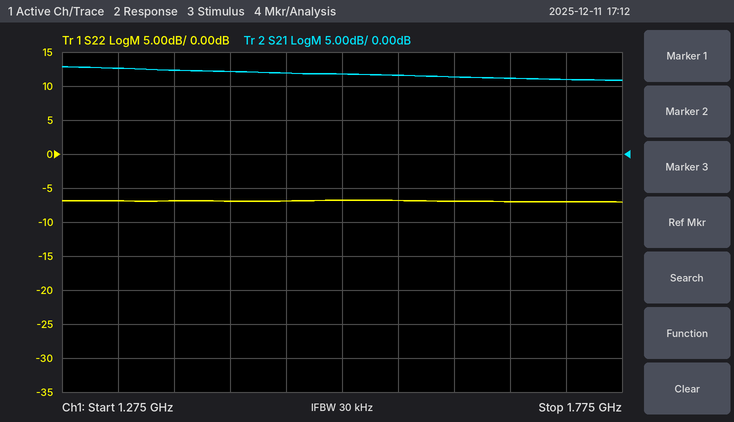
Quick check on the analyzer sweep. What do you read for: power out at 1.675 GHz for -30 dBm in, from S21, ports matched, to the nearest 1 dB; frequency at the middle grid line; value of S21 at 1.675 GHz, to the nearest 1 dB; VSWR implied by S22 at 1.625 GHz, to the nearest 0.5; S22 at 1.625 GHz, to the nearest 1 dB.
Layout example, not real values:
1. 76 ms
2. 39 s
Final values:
1. -19 dBm
2. 1.525 GHz
3. 11 dB
4. 2.5
5. -7 dB
